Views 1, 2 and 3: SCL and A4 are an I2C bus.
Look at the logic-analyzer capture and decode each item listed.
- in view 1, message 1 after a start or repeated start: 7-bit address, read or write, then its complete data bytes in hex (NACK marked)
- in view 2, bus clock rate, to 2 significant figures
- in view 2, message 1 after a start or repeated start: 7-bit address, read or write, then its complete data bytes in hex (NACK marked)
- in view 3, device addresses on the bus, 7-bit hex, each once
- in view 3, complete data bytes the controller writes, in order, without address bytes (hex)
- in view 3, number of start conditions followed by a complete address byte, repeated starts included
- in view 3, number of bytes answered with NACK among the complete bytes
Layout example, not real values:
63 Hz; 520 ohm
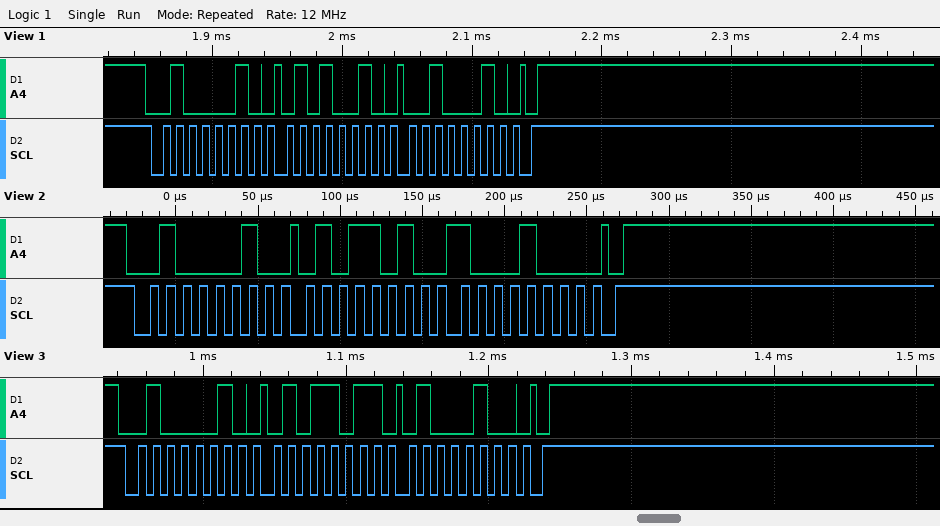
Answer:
0x21 write: 52 22; 100 kHz; 0x21 write: 5A 88; 0x21; 5B 44; 1; 0
